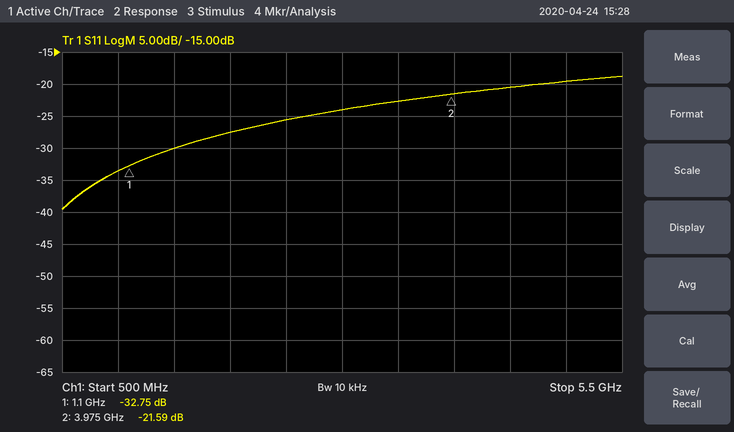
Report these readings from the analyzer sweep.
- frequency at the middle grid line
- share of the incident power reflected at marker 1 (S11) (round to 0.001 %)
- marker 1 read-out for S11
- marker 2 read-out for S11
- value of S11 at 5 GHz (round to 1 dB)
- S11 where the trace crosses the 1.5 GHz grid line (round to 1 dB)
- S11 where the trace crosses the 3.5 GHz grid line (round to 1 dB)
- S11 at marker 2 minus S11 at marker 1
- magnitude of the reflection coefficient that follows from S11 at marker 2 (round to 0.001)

3 GHz
0.053 %
-32.75 dB
-21.59 dB
-20 dB
-30 dB
-23 dB
11.16 dB
0.083
